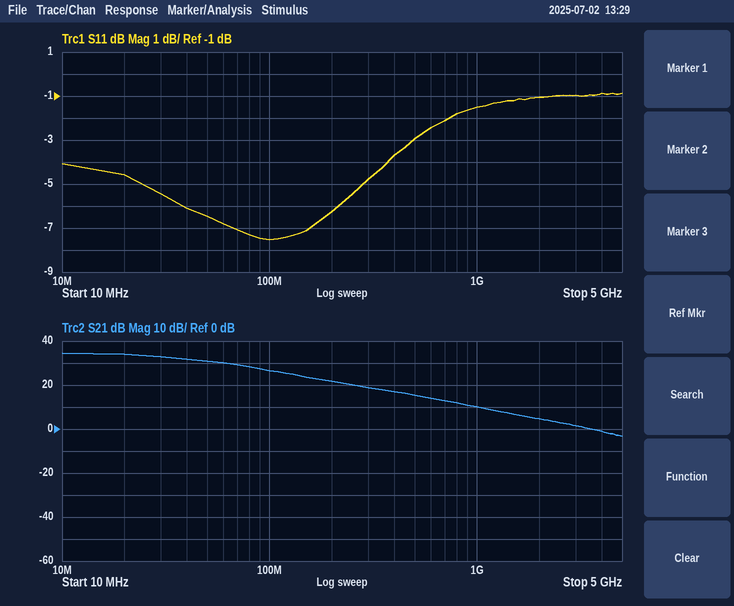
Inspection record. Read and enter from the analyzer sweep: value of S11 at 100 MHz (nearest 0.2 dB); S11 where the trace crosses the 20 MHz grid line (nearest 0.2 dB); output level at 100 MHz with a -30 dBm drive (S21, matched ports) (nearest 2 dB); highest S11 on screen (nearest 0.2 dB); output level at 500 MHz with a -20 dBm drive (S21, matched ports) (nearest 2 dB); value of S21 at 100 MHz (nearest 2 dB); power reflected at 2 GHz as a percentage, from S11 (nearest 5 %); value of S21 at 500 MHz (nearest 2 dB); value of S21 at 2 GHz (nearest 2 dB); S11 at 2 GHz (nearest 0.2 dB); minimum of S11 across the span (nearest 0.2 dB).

-7.6 dB
-4.6 dB
-4 dBm
-0.8 dB
-4 dBm
26 dB
80 %
16 dB
4 dB
-1.0 dB
-7.6 dB
